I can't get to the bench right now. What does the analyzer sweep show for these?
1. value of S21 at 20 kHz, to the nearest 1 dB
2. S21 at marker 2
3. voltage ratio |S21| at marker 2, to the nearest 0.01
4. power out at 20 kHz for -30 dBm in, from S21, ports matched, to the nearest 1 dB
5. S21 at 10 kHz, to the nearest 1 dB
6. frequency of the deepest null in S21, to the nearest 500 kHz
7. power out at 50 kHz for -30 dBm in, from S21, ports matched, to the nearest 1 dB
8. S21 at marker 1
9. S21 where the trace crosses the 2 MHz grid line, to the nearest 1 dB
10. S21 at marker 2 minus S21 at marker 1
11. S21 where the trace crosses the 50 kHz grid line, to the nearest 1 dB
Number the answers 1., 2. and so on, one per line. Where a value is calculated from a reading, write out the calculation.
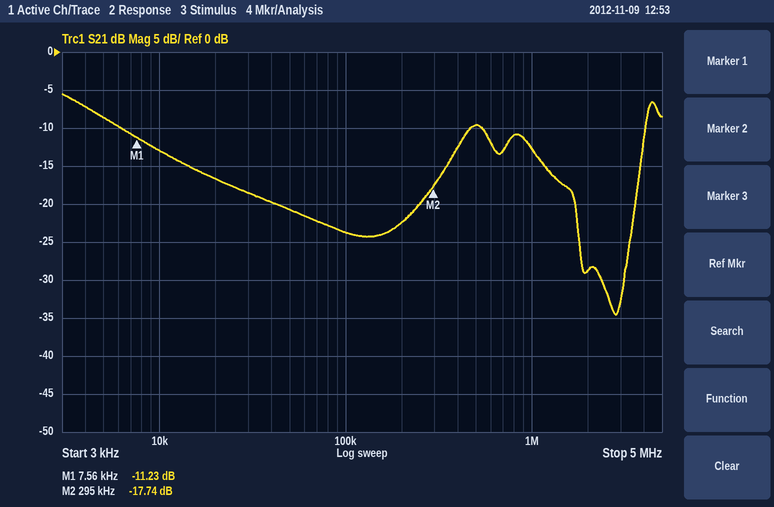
1. -17 dB
2. -17.74 dB
3. 10^(-17.74/20) ≈ 0.13
4. -30 dBm + (-17 dB) = -47 dBm
5. -13 dB
6. 3.0 MHz
7. -30 dBm + (-21 dB) = -51 dBm
8. -11.23 dB
9. -29 dB
10. -17.74 − (-11.23) = -6.51 dB
11. -21 dB
